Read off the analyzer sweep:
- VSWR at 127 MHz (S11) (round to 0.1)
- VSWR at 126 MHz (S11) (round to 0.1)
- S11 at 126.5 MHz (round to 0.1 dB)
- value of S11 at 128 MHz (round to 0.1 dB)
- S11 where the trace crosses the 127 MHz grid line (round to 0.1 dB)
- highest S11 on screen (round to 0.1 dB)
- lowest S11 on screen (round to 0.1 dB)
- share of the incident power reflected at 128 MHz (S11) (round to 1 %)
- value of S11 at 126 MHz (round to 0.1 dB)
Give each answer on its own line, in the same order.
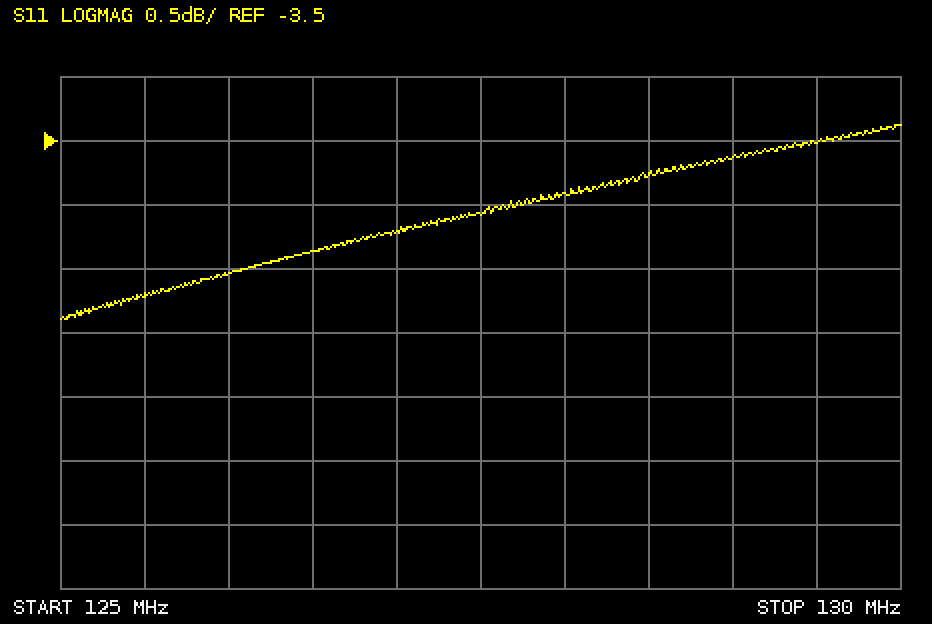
4.2
3.9
-4.4 dB
-3.9 dB
-4.2 dB
-3.4 dB
-4.9 dB
41 %
-4.5 dB
